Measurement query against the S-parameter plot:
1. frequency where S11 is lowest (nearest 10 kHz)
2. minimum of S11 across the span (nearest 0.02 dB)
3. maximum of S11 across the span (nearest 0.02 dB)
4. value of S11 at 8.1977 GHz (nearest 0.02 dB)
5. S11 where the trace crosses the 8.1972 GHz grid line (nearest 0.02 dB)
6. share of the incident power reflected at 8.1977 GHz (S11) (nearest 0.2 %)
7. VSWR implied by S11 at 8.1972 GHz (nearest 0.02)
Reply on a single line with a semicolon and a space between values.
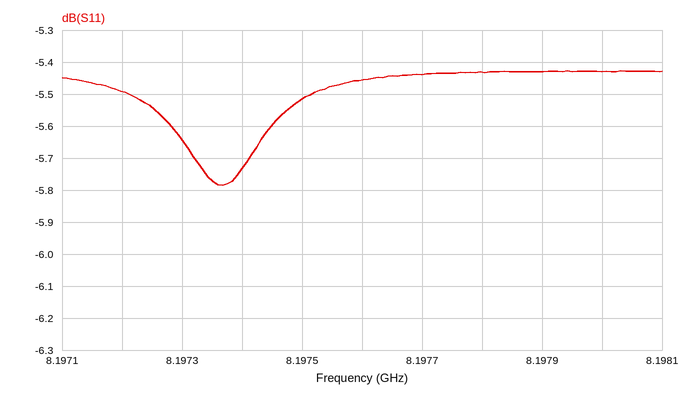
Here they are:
8.19737 GHz; -5.78 dB; -5.42 dB; -5.44 dB; -5.50 dB; 28.6 %; 3.26
